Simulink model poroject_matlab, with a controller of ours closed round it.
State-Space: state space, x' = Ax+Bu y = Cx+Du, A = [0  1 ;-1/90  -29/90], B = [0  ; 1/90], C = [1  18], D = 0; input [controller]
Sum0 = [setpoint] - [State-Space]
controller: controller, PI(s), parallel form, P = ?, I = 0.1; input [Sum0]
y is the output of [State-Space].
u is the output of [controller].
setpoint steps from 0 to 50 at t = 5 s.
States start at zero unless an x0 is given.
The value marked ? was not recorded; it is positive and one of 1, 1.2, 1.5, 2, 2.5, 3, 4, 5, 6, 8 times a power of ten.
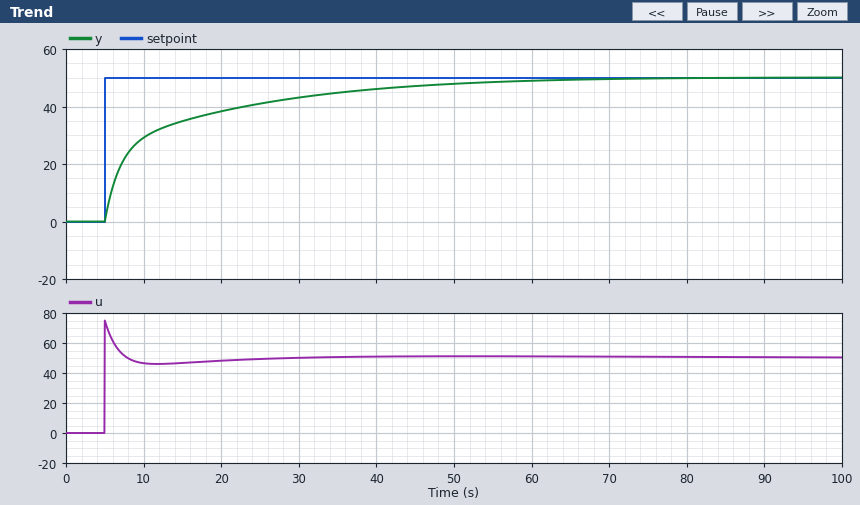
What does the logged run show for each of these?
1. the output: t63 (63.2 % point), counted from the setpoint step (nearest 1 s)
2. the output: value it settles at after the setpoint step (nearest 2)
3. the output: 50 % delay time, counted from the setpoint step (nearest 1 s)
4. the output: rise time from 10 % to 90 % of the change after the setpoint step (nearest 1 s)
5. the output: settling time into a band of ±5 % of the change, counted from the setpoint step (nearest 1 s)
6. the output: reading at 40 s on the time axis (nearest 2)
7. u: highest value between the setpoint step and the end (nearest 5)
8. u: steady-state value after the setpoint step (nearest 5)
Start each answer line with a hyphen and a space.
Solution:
- 7 s
- 50
- 3 s
- 30 s
- 42 s
- 46
- 75
- 50
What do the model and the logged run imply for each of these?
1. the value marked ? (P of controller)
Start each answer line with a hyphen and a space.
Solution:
- 1.5
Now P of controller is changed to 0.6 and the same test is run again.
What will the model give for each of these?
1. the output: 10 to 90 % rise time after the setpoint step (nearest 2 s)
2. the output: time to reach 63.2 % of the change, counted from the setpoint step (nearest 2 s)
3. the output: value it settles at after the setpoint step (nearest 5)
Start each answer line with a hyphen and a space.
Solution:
- 26 s
- 12 s
- 50
